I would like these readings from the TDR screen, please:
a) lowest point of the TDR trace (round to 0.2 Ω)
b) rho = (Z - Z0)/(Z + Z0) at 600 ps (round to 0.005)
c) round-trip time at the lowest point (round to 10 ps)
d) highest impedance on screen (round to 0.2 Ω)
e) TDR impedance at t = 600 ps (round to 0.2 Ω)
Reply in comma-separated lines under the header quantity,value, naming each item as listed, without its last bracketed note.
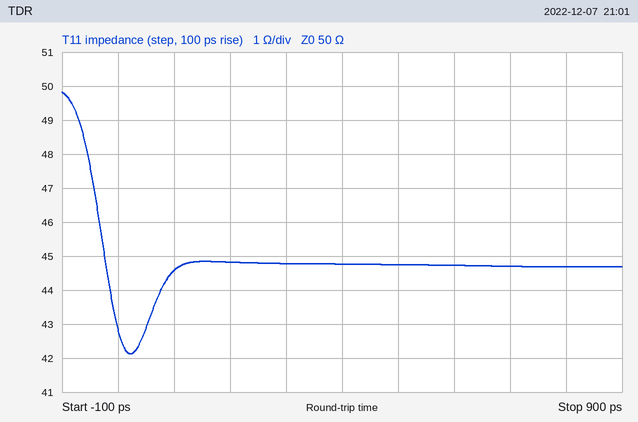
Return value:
quantity,value
lowest point of the TDR trace,42.2 Ω
rho = (Z - Z0)/(Z + Z0) at 600 ps,-0.055
round-trip time at the lowest point,20 ps
highest impedance on screen,49.8 Ω
TDR impedance at t = 600 ps,44.8 Ω
